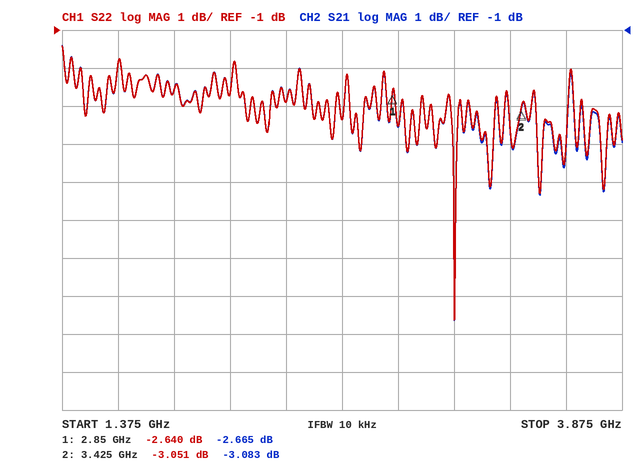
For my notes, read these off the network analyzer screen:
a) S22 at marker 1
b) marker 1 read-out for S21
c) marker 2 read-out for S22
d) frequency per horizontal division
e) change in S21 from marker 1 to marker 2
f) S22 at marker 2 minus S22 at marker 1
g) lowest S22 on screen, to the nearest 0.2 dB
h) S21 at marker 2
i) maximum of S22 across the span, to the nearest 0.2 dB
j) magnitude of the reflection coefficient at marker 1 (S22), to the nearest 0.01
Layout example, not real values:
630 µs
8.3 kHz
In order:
-2.640 dB
-2.665 dB
-3.051 dB
250 MHz
-0.418 dB
-0.411 dB
-8.6 dB
-3.083 dB
-1.4 dB
0.74
